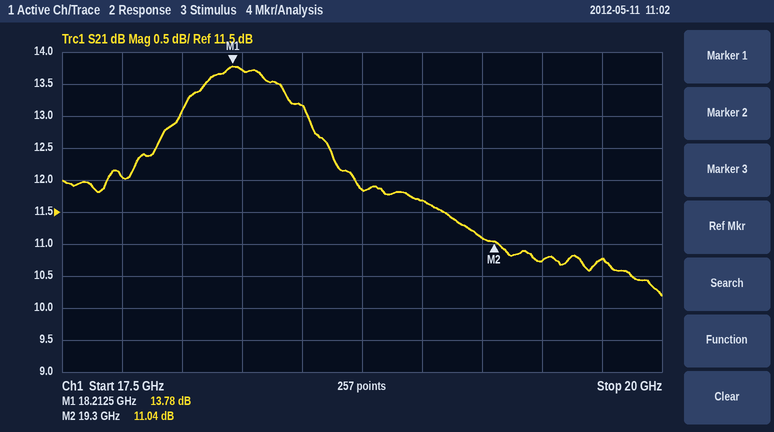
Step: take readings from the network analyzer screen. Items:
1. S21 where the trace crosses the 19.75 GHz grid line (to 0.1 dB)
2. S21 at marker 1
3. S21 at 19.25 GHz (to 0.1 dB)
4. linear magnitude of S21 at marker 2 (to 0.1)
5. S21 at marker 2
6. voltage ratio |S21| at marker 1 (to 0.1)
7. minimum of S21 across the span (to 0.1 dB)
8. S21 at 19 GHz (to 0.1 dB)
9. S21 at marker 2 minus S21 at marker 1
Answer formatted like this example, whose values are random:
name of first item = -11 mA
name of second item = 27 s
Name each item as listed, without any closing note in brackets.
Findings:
S21 where the trace crosses the 19.75 GHz grid line = 10.8 dB
S21 at marker 1 = 13.78 dB
S21 at 19.25 GHz = 11.1 dB
linear magnitude of S21 at marker 2 = 3.6
S21 at marker 2 = 11.04 dB
voltage ratio |S21| at marker 1 = 4.9
minimum of S21 across the span = 10.2 dB
S21 at 19 GHz = 11.7 dB
S21 at marker 2 minus S21 at marker 1 = -2.74 dB
